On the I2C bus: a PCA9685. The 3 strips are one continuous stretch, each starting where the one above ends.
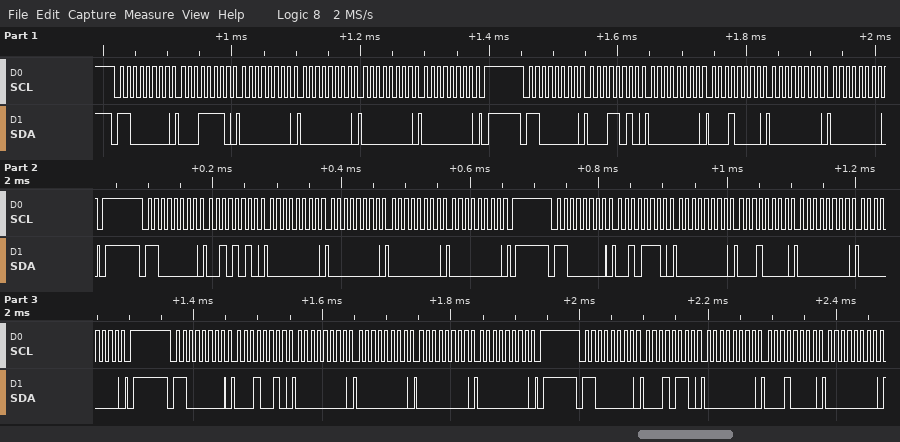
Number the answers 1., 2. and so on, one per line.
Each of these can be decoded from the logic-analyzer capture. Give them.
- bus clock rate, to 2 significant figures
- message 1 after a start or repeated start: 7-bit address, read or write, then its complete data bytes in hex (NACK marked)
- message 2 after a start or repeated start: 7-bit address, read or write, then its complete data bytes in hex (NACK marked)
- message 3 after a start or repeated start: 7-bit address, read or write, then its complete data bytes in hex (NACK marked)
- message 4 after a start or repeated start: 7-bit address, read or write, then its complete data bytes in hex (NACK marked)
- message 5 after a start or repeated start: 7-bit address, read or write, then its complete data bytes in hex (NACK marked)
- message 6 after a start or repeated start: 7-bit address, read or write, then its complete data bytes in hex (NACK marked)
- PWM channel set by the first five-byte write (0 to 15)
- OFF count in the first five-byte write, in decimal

1. 100 kHz
2. 0x60 write: 1E 00 00 00 00
3. 0x60 write: 1A 00 10 00 00
4. 0x60 write: 2A 00 00 00 00
5. 0x60 write: 2E 00 10 00 00
6. 0x60 write: 12 00 00 00 00
7. 0x60 write: 16 00 10 00
8. 6
9. 0
